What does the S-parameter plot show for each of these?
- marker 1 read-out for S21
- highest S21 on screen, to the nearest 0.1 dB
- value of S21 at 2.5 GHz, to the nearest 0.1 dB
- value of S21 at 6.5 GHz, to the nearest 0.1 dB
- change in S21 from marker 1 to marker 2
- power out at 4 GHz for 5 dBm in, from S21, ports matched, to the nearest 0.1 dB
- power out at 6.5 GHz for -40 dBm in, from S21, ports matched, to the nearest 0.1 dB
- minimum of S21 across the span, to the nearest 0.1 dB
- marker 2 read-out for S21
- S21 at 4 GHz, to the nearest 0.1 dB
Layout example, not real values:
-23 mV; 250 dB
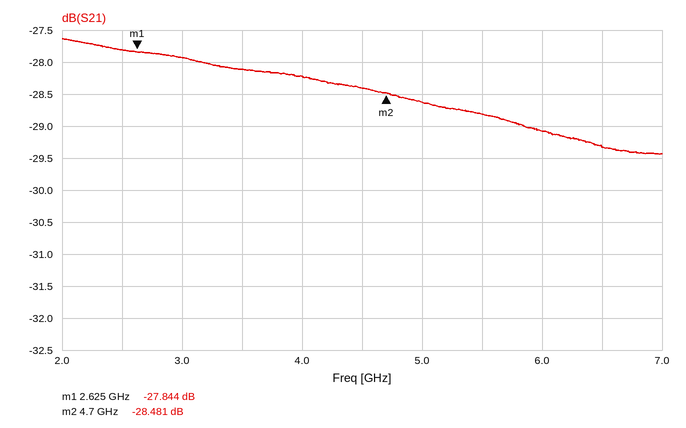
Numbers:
-27.844 dB; -27.6 dB; -27.8 dB; -29.3 dB; -0.637 dB; -23.2 dBm; -69.3 dBm; -29.4 dB; -28.481 dB; -28.2 dB
